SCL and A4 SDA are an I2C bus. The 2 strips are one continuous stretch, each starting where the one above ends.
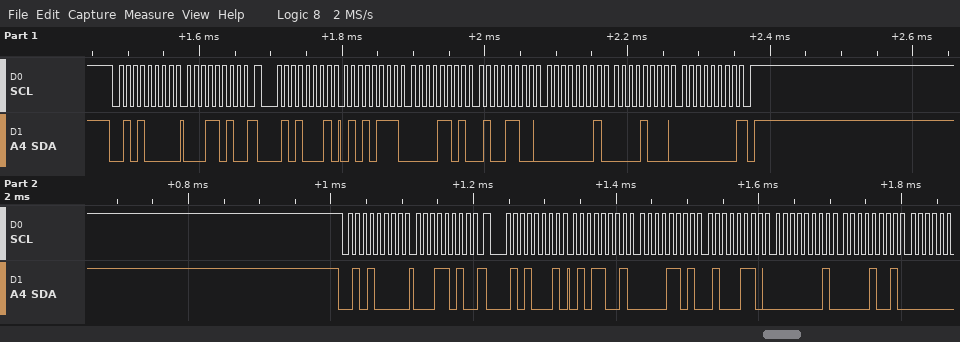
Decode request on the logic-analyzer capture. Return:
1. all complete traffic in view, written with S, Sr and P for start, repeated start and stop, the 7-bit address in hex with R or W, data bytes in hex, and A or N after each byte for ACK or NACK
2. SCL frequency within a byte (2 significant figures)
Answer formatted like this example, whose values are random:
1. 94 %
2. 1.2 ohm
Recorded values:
1. S 28W A 1A A Sr 28R A 57 A 0D A 4C A 01 A 08 A 00 N P S 28W A 1A A Sr 28R A 59 A 0D A 46 A 01 A 09 A
2. 100 kHz
